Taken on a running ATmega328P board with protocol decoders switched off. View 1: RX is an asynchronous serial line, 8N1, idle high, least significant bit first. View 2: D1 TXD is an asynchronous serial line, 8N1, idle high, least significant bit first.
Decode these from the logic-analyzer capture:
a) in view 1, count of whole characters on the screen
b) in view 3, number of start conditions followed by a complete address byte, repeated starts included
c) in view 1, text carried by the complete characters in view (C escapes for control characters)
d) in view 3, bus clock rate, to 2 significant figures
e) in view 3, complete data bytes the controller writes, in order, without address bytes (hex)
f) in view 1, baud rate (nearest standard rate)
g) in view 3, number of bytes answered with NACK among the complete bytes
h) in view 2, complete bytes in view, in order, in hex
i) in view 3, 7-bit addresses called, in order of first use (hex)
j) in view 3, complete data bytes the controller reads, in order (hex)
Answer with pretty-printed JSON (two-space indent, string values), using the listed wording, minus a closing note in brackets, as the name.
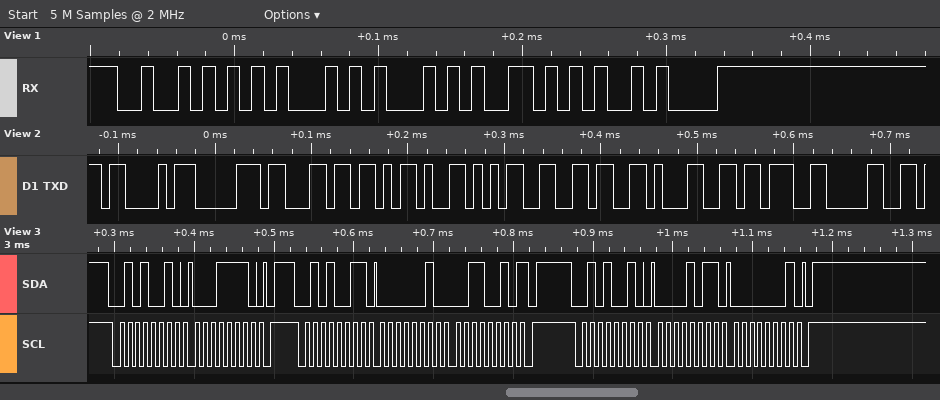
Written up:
{
  "in view 1, count of whole characters on the screen": "5",
  "in view 3, number of start conditions followed by a complete address byte, repeated starts included": "3",
  "in view 1, text carried by the complete characters in view": "\"REQV\\n\"",
  "in view 3, bus clock rate, to 2 significant figures": "100 kHz",
  "in view 3, complete data bytes the controller writes, in order, without address bytes": "1E 0B 01",
  "in view 1, baud rate": "115200 baud",
  "in view 3, number of bytes answered with NACK among the complete bytes": "1",
  "in view 2, complete bytes in view, in order, in hex": "43 70 6C 2D 35 36 31 3B 30",
  "in view 3, 7-bit addresses called, in order of first use": "0x29",
  "in view 3, complete data bytes the controller reads, in order": "02 32"
}
